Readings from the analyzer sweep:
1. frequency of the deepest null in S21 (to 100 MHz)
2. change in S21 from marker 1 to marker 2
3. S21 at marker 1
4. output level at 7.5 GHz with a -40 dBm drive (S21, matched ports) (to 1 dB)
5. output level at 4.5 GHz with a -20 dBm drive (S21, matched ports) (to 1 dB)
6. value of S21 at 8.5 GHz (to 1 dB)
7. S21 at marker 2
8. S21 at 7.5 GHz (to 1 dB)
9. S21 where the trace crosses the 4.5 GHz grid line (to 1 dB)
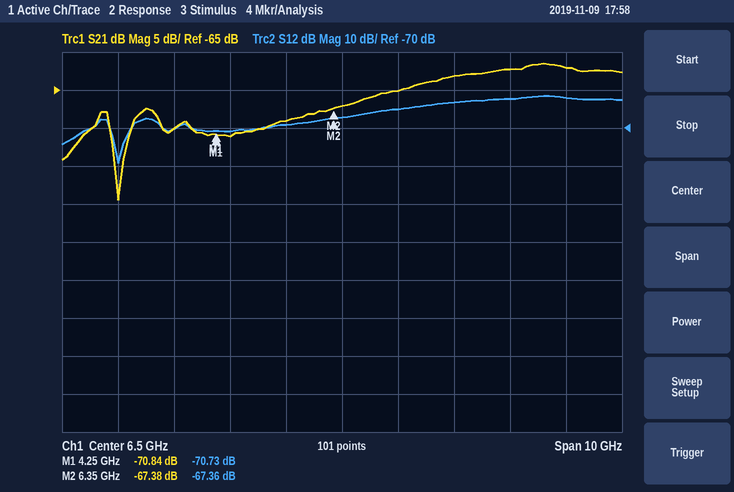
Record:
2.5 GHz
3.46 dB
-70.84 dB
-105 dBm
-91 dBm
-63 dB
-67.38 dB
-65 dB
-71 dB
